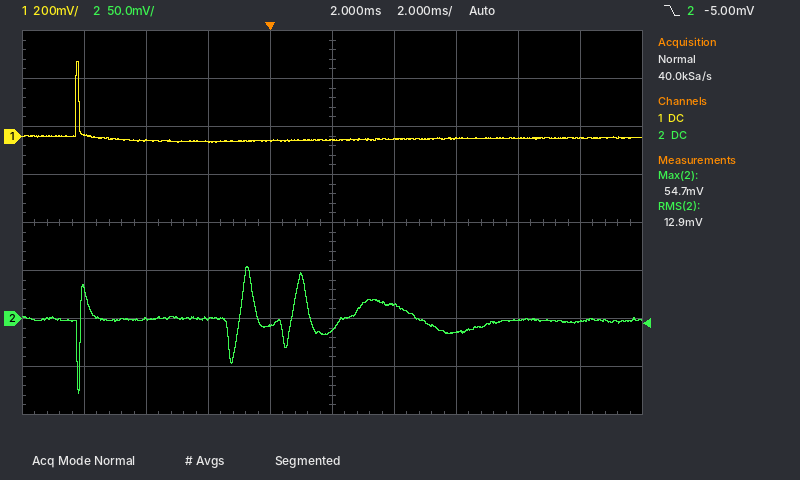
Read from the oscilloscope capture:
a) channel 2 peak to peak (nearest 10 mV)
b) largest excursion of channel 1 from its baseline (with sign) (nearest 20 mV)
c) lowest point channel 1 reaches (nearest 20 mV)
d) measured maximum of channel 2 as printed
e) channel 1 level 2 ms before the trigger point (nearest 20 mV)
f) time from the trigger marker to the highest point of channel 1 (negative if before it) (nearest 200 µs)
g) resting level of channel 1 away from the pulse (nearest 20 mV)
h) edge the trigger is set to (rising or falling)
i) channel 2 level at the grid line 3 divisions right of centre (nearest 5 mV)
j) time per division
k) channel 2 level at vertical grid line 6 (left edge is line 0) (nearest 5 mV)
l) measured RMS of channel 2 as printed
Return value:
130 mV
+320 mV
-20 mV
54.7 mV
-20 mV
-6.2 ms
-20 mV
falling
0 mV
2 ms
15 mV
12.9 mV
